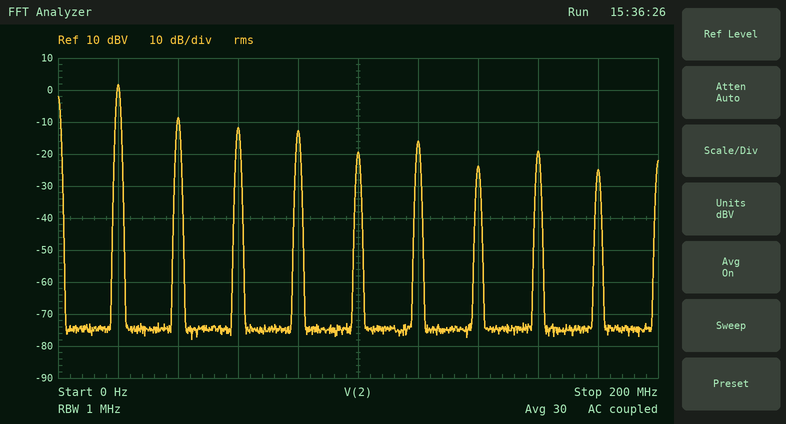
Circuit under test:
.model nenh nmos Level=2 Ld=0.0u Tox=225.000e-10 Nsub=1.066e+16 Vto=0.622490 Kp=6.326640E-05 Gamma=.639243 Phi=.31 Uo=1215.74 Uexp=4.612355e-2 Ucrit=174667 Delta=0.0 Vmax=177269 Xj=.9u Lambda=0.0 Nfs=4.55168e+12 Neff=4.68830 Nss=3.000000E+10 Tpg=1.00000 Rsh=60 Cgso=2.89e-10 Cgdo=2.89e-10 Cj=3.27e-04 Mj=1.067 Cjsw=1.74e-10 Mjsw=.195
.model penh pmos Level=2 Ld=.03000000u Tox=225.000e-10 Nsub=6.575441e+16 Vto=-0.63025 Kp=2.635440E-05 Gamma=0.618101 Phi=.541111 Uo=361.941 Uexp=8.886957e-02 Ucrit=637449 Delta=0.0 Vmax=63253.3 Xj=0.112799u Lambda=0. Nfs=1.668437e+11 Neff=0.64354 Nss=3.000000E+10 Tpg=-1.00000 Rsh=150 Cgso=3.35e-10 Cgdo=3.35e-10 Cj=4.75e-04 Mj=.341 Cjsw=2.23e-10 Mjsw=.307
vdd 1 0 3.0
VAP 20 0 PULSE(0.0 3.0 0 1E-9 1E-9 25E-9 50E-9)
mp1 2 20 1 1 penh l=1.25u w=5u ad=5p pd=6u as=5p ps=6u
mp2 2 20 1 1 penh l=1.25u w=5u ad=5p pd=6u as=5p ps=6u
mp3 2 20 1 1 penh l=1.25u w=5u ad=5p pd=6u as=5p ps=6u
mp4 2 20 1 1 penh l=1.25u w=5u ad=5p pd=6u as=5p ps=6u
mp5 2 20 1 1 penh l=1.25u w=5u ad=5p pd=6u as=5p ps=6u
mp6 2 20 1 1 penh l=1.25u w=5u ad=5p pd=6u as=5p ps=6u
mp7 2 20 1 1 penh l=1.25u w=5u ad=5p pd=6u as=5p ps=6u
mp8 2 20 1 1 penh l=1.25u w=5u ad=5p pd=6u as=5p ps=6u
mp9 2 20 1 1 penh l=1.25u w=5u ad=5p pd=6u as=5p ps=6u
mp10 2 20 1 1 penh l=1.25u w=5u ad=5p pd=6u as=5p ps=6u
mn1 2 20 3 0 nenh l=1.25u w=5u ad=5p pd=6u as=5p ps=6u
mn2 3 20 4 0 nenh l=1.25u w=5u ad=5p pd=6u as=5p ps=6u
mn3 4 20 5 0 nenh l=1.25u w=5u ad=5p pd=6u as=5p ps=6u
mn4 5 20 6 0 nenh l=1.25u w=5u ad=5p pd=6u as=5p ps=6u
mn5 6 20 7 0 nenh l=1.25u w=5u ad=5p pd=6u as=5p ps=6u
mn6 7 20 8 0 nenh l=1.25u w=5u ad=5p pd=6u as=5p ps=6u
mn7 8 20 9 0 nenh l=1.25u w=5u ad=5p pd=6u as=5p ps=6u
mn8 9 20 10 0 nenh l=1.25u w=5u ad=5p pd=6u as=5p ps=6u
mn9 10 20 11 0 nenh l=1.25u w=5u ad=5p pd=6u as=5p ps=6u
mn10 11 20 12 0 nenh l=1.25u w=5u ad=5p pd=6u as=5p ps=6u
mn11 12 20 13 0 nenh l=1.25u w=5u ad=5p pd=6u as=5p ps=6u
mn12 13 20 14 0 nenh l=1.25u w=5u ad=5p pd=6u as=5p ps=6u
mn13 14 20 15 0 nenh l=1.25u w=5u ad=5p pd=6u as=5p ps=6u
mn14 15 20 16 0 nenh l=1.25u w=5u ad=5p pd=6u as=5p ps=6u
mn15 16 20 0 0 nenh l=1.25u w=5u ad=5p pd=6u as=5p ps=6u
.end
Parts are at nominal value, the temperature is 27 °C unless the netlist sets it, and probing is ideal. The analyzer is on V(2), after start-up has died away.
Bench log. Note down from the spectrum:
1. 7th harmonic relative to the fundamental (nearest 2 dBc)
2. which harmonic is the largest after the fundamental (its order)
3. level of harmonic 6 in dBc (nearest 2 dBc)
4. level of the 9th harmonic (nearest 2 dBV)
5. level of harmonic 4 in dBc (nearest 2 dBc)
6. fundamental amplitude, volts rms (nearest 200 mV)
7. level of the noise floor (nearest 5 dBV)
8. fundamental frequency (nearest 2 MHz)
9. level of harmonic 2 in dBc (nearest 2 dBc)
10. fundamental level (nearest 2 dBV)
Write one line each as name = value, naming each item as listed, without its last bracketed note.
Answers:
7th harmonic relative to the fundamental = -26 dBc
which harmonic is the largest after the fundamental = 2
level of harmonic 6 in dBc = -18 dBc
level of the 9th harmonic = -24 dBV
level of harmonic 4 in dBc = -14 dBc
fundamental amplitude, volts rms = 1.2 V
level of the noise floor = -75 dBV
fundamental frequency = 20 MHz
level of harmonic 2 in dBc = -10 dBc
fundamental level = 2 dBV
